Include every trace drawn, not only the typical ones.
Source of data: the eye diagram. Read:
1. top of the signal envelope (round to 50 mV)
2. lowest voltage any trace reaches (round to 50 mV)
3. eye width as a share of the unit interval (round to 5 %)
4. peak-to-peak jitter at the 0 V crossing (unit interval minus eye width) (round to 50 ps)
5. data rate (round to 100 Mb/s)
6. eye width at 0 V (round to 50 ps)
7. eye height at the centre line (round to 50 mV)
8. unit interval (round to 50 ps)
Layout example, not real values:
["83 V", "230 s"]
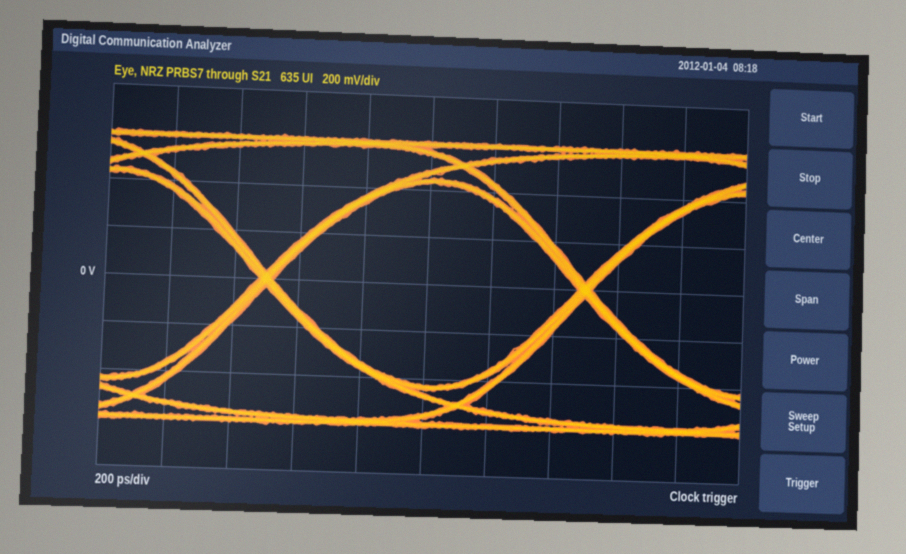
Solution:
["600 mV", "-600 mV", "95 %", "50 ps", "1.0 Gb/s", "950 ps", "850 mV", "1.00 ns"]
